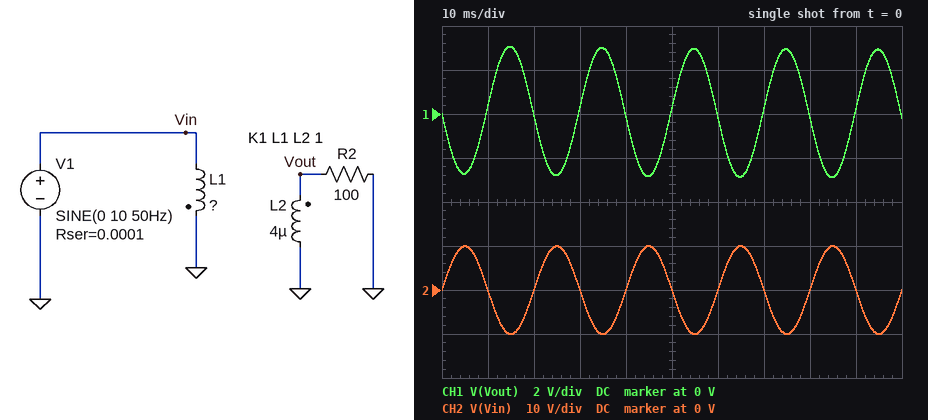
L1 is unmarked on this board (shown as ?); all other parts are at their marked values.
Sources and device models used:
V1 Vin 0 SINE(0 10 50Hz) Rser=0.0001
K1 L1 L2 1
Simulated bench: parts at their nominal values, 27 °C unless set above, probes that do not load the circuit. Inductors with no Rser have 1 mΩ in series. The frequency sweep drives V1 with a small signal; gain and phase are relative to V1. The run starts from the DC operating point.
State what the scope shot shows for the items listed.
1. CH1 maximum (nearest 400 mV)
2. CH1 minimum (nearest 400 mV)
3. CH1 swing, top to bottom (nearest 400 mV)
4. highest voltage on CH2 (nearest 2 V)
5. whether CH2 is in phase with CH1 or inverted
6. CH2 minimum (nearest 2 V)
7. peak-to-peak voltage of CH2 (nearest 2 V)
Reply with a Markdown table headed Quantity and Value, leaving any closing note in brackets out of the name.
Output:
| Quantity | Value |
|---|---|
| CH1 maximum | 3.2 V |
| CH1 minimum | -2.8 V |
| CH1 swing, top to bottom | 6.0 V |
| highest voltage on CH2 | 10 V |
| whether CH2 is in phase with CH1 or inverted | inverted |
| CH2 minimum | -10 V |
| peak-to-peak voltage of CH2 | 20 V |
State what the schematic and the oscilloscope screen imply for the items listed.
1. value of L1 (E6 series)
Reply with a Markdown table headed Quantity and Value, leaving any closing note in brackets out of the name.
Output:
| Quantity | Value |
|---|---|
| value of L1 | 47 µH |
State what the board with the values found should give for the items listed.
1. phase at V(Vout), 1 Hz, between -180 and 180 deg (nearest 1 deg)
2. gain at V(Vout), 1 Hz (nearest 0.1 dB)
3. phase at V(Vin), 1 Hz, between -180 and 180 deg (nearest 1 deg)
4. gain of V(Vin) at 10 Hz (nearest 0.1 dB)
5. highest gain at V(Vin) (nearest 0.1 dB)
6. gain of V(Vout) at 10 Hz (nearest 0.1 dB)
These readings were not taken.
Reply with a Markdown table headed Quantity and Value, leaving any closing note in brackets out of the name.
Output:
| Quantity | Value |
|---|---|
| phase at V(Vout), 1 Hz, between -180 and 180 deg | -105 deg |
| gain at V(Vout), 1 Hz | -22.4 dB |
| phase at V(Vin), 1 Hz, between -180 and 180 deg | 1 deg |
| gain of V(Vin) at 10 Hz | -0.1 dB |
| highest gain at V(Vin) | 0 dB |
| gain of V(Vout) at 10 Hz | -11.3 dB |
